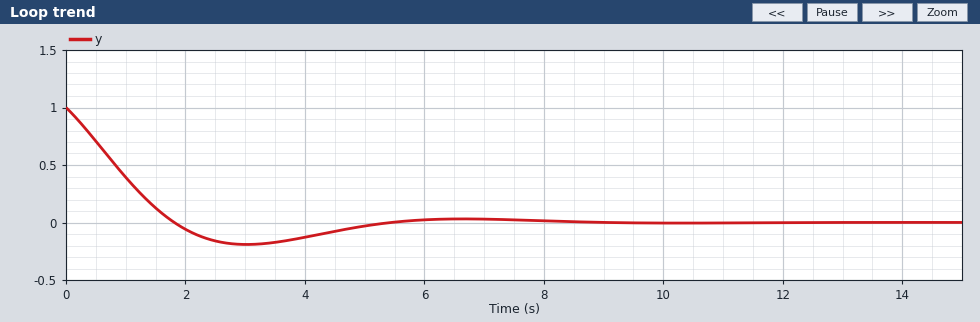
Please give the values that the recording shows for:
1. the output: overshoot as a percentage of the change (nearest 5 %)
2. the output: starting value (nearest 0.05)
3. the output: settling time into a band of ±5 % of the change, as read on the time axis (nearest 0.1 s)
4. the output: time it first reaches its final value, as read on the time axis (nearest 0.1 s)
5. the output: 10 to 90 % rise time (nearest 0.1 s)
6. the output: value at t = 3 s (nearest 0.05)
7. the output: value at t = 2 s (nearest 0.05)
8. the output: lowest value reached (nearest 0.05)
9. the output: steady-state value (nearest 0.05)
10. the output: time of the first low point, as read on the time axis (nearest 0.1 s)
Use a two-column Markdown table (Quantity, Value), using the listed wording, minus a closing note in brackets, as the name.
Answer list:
| Quantity | Value |
|---|---|
| the output: overshoot as a percentage of the change | 20 % |
| the output: starting value | 1.00 |
| the output: settling time into a band of ±5 % of the change, as read on the time axis | 4.8 s |
| the output: time it first reaches its final value, as read on the time axis | 1.8 s |
| the output: 10 to 90 % rise time | 1.4 s |
| the output: value at t = 3 s | -0.20 |
| the output: value at t = 2 s | -0.05 |
| the output: lowest value reached | -0.20 |
| the output: steady-state value | 0.00 |
| the output: time of the first low point, as read on the time axis | 3.0 s |
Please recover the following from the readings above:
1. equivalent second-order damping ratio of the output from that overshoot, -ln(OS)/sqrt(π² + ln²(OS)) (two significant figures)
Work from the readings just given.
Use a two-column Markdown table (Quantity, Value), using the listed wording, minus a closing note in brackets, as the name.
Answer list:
| Quantity | Value |
|---|---|
| equivalent second-order damping ratio of the output from that overshoot, -ln(OS)/sqrt(π² + ln²(OS)) | 0.46 |
